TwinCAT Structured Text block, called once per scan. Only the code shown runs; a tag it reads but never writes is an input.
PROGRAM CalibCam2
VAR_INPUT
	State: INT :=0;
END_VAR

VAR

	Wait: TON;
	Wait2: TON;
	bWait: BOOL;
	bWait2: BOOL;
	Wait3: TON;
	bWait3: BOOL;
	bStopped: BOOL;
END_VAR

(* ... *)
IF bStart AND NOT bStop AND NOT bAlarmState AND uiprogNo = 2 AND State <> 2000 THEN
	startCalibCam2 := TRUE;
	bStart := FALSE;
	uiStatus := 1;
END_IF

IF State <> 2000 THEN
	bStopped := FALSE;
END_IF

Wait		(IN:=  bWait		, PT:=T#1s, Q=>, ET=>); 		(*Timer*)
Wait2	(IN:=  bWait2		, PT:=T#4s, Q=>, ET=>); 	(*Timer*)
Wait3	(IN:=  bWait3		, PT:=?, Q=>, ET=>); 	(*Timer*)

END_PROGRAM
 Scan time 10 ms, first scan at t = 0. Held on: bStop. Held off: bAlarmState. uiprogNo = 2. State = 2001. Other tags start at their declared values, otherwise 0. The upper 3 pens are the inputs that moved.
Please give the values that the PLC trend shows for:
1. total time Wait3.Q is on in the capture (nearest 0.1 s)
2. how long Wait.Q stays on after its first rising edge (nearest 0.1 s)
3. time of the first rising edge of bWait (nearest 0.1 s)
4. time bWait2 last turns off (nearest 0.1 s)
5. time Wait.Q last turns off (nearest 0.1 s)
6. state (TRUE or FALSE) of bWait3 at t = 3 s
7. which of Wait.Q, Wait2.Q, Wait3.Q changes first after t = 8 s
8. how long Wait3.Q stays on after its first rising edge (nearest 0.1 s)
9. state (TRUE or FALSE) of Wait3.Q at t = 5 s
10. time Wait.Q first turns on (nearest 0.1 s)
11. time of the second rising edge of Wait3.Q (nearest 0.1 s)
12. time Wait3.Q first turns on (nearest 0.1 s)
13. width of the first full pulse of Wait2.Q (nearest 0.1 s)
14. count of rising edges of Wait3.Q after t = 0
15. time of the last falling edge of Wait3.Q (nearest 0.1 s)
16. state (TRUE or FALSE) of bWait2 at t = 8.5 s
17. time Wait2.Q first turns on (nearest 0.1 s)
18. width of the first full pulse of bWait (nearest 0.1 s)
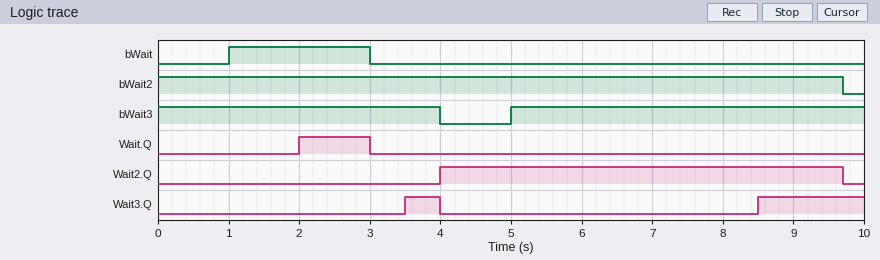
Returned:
2.0 s
1.0 s
1.0 s
9.7 s
3.0 s
TRUE
Wait3.Q
0.5 s
FALSE
2.0 s
8.5 s
3.5 s
5.7 s
2
4.0 s
TRUE
4.0 s
2.0 s
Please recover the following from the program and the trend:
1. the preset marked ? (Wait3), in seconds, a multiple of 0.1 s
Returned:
3.5 s
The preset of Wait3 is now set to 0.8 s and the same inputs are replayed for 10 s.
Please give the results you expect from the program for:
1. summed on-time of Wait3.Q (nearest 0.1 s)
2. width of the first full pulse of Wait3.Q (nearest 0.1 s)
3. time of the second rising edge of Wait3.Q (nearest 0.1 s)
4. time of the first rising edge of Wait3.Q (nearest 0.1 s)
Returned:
7.4 s
3.2 s
5.8 s
0.8 s
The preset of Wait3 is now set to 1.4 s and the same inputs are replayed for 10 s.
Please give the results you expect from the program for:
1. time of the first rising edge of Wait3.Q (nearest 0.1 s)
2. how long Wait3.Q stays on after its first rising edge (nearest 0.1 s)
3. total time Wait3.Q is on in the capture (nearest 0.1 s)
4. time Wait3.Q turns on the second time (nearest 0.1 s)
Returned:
1.4 s
2.6 s
6.2 s
6.4 s
